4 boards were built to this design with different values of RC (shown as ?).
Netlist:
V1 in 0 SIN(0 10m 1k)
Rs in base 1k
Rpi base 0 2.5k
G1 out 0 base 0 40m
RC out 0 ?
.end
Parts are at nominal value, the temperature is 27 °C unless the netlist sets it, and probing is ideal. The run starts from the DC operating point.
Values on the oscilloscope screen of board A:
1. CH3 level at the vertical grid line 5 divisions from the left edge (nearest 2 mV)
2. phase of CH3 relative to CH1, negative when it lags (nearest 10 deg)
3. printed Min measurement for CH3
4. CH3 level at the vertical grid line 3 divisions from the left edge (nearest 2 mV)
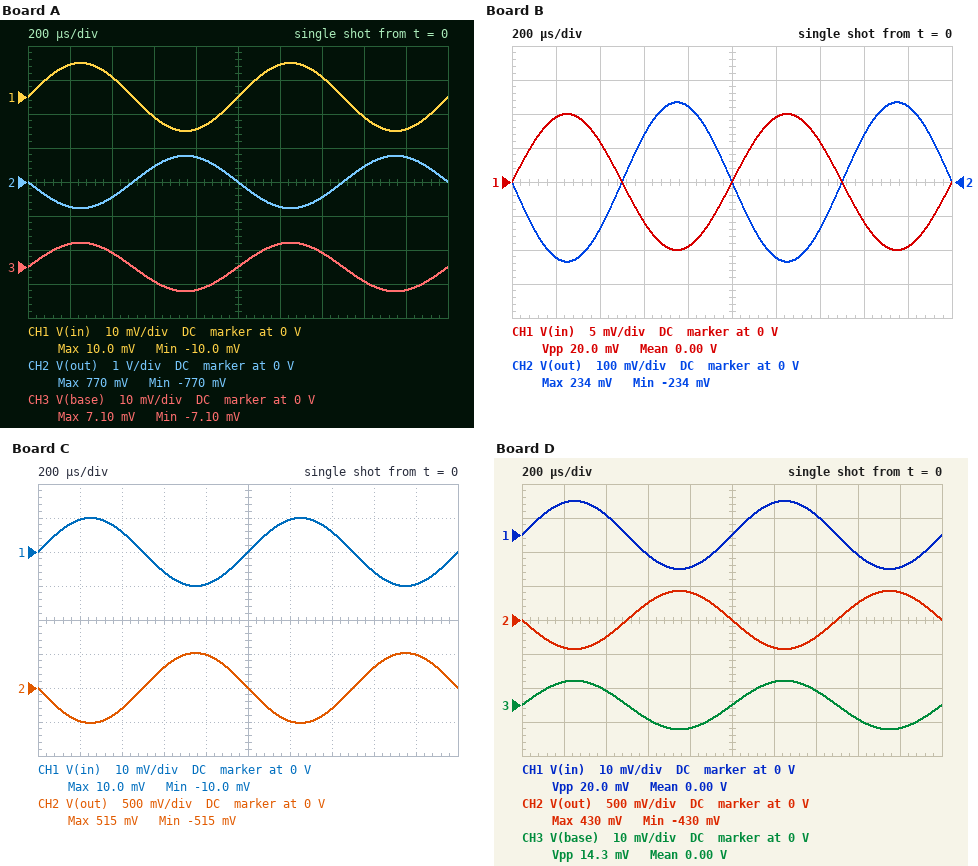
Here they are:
0 V
0 deg
-7.10 mV
-4 mV
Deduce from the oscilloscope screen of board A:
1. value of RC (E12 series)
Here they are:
2.7 kΩ
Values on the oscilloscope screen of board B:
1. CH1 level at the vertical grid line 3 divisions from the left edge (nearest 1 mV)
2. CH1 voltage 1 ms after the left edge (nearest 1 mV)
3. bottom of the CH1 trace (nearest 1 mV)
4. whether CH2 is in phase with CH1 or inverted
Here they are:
-6 mV
0 V
-10 mV
inverted
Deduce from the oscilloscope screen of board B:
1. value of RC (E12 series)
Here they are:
820 Ω
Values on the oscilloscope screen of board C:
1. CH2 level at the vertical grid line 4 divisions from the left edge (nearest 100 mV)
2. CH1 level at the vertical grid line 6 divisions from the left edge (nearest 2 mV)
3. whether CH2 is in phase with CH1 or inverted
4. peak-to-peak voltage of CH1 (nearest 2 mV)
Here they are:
500 mV
10 mV
inverted
20 mV
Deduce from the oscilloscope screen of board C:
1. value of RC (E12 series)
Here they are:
1.8 kΩ
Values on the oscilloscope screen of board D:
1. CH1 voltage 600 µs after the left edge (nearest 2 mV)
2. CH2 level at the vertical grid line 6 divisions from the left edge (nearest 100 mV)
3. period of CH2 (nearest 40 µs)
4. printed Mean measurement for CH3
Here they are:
-6 mV
-400 mV
1.00 ms
0.00 V
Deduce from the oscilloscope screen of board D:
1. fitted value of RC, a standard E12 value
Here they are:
1.5 kΩ
